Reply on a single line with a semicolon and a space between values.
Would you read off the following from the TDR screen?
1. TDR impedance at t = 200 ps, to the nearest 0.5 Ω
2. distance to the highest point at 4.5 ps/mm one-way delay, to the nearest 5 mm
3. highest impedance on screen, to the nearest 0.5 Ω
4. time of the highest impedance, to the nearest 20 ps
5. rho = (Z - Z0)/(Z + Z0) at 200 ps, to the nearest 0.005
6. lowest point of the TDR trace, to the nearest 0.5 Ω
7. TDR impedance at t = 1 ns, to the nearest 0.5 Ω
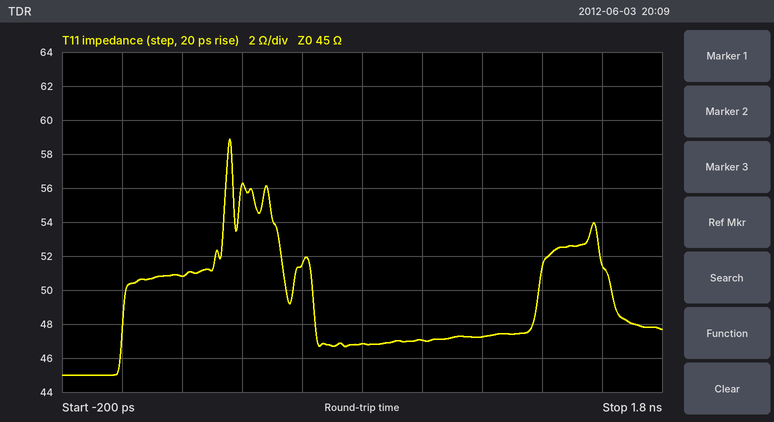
51.0 Ω; 40 mm; 59.0 Ω; 360 ps; +0.060; 45.0 Ω; 47.0 Ω
